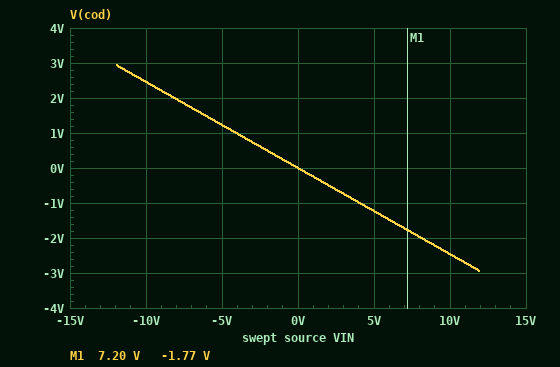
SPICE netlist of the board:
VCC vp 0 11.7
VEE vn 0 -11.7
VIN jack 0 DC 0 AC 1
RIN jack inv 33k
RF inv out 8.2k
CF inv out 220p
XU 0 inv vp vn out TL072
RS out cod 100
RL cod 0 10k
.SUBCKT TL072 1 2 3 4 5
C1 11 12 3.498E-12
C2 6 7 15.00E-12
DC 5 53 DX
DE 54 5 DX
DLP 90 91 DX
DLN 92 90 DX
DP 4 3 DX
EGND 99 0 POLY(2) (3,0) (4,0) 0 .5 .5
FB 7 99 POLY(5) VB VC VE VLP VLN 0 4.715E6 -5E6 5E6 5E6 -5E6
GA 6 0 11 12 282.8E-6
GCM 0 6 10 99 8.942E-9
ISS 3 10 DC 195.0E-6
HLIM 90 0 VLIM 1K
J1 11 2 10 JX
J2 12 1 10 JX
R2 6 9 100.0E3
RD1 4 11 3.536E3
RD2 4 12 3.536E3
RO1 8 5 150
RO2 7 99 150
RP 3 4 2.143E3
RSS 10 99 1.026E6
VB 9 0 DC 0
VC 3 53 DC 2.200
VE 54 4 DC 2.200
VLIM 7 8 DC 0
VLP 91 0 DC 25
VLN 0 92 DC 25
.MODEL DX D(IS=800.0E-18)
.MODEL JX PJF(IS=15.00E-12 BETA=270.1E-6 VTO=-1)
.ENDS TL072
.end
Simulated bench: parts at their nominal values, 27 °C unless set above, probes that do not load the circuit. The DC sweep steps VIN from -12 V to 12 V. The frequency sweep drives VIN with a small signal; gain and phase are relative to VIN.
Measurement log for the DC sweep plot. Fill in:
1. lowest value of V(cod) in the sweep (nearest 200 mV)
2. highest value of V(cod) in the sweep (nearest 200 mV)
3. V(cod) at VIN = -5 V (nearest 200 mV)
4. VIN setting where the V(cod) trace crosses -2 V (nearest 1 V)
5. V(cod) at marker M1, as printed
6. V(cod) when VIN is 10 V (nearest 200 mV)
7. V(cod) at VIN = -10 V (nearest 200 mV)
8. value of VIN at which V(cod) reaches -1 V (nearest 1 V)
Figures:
-3.0 V
3.0 V
1.2 V
8 V
-1.77 V
-2.4 V
2.4 V
4 V
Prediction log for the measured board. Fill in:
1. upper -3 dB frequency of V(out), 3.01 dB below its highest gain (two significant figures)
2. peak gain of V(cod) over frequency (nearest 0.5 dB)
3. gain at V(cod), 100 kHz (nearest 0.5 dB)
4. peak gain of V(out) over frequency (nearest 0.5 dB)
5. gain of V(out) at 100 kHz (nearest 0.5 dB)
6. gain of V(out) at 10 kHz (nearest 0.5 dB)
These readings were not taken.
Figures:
88 kHz
-12.0 dB
-16.0 dB
-12.0 dB
-15.5 dB
-12.0 dB
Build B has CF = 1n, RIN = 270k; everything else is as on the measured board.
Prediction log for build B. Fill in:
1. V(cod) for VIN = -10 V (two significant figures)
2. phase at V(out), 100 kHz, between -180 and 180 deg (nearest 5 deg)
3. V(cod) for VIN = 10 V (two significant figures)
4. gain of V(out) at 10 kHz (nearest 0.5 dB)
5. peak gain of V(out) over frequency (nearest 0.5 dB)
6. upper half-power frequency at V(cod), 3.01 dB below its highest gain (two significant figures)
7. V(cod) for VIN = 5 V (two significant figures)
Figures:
300 mV
100 deg
-300 mV
-31.5 dB
-30.5 dB
19 kHz
-150 mV
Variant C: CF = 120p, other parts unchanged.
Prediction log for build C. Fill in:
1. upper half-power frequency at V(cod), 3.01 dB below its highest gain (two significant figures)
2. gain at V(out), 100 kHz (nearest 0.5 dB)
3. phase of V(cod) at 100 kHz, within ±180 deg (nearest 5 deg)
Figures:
160 kHz
-13.5 dB
145 deg
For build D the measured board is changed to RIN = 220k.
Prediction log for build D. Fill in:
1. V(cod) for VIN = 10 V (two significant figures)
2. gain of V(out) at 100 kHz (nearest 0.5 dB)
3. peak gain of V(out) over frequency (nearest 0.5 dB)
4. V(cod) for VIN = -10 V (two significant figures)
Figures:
-370 mV
-32.0 dB
-28.5 dB
370 mV
